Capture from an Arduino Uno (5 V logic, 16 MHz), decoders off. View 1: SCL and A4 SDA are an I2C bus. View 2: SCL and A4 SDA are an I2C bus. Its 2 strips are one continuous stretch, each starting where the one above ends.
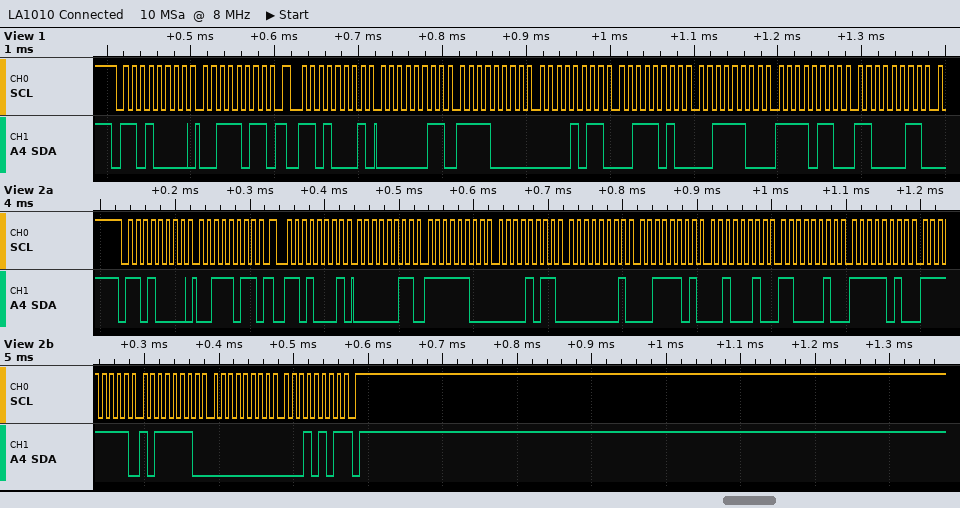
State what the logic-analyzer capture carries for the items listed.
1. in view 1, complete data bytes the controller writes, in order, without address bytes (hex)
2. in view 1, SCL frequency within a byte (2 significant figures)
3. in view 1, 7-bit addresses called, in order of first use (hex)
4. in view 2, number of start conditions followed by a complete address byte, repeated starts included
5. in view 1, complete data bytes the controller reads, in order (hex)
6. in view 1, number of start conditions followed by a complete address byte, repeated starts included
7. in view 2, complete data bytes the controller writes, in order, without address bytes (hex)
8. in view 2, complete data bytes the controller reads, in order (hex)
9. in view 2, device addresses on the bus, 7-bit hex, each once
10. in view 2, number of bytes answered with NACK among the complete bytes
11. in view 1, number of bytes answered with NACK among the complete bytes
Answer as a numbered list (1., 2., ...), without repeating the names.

1. 3B
2. 100 kHz
3. 0x68
4. 2
5. 03 F0 0B 3A 3C F6 C3
6. 2
7. 3B
8. 03 FC 0B 01 3D 22 C2 FA FF BE 00 15
9. 0x68
10. 1
11. 0
